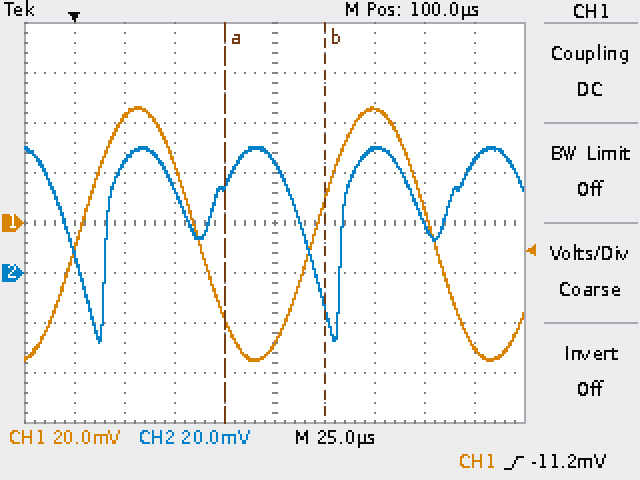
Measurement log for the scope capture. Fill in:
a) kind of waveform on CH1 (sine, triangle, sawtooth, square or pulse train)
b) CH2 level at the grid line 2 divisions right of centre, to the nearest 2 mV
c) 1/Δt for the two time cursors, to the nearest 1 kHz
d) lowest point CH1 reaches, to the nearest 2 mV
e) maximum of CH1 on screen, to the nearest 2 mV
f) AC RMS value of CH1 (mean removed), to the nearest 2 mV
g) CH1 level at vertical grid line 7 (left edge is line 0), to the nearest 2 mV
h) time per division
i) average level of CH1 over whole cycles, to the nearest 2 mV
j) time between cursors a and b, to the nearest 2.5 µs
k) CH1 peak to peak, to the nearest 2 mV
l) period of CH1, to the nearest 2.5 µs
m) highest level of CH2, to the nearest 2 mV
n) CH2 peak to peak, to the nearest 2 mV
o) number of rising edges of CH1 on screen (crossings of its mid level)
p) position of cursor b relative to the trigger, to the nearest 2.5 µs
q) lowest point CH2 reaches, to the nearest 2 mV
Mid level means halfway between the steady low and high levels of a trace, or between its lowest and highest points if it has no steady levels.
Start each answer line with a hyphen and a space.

- sine
- 50 mV
- 20 kHz
- -56 mV
- 46 mV
- 36 mV
- 46 mV
- 25 µs
- -4 mV
- 50.0 µs
- 102 mV
- 117.5 µs
- 50 mV
- 78 mV
- 2
- +125.0 µs
- -28 mV
